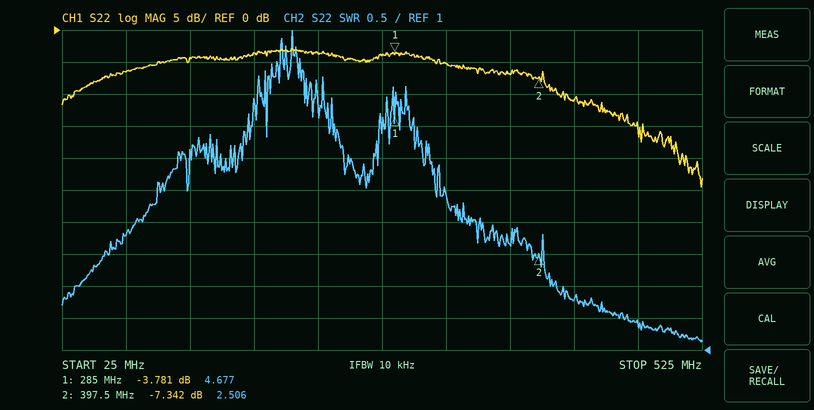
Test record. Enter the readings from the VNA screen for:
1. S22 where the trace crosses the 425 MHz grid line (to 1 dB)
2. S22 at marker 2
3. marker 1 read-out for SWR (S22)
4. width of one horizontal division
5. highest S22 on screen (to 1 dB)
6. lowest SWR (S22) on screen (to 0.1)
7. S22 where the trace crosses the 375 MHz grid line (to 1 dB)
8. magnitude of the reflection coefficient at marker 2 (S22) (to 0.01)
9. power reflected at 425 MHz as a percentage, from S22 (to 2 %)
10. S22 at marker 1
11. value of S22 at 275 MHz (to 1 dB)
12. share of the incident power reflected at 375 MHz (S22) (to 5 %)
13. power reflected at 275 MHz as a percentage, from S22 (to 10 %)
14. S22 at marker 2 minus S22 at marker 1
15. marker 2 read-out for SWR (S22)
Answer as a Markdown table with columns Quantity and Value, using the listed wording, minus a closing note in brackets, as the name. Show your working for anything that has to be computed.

| Quantity | Value |
|---|---|
| S22 where the trace crosses the 425 MHz grid line | -11 dB |
| S22 at marker 2 | -7.342 dB |
| marker 1 read-out for SWR | 4.677 |
| width of one horizontal division | 50 MHz |
| highest S22 on screen | -3 dB |
| lowest SWR (S22) on screen | 1.1 |
| S22 where the trace crosses the 375 MHz grid line | -7 dB |
| magnitude of the reflection coefficient at marker 2 (S22) | 10^(-7.342/20) ≈ 0.43 |
| power reflected at 425 MHz as a percentage, from S22 | 10^(-11/10) ≈ 8 % |
| S22 at marker 1 | -3.781 dB |
| value of S22 at 275 MHz | -4 dB |
| share of the incident power reflected at 375 MHz (S22) | 10^(-7/10) ≈ 20 % |
| power reflected at 275 MHz as a percentage, from S22 | 10^(-4/10) ≈ 40 % |
| S22 at marker 2 minus S22 at marker 1 | -7.342 − (-3.781) = -3.561 dB |
| marker 2 read-out for SWR | 2.506 |
